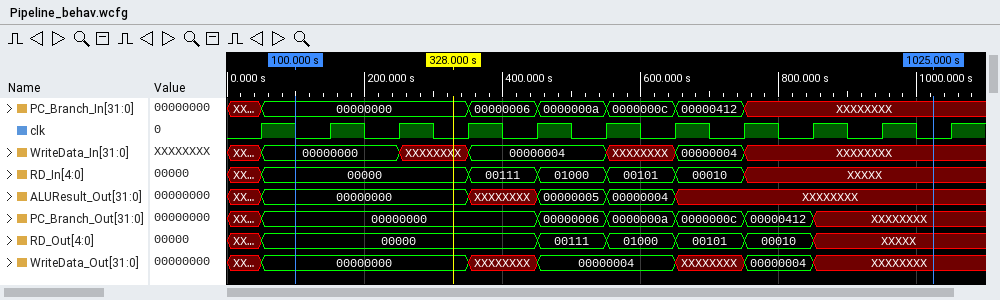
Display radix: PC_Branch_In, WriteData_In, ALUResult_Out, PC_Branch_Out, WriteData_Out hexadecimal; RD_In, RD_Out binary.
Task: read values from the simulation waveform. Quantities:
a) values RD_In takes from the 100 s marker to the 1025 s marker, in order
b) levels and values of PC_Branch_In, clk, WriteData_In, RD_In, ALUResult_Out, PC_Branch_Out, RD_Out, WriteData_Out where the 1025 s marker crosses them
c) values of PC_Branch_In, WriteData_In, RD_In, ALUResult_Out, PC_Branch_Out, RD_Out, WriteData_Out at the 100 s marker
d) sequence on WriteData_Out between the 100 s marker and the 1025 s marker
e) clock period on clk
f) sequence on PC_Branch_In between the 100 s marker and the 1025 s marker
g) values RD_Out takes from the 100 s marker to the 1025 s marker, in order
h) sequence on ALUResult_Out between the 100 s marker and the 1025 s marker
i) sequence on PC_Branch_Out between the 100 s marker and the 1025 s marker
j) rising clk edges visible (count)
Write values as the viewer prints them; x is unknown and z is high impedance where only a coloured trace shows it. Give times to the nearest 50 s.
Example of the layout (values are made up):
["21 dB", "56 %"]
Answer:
["00000, 00111, 01000, 00101, 00010, XXXXX", "PC_Branch_In=XXXXXXXX, clk=0, WriteData_In=XXXXXXXX, RD_In=XXXXX, ALUResult_Out=XXXXXXXX, PC_Branch_Out=XXXXXXXX, RD_Out=XXXXX, WriteData_Out=XXXXXXXX", "PC_Branch_In=00000000, WriteData_In=00000000, RD_In=00000, ALUResult_Out=00000000, PC_Branch_Out=00000000, RD_Out=00000, WriteData_Out=00000000", "00000000, XXXXXXXX, 00000004, XXXXXXXX, 00000004, XXXXXXXX", "100 s", "00000000, 00000006, 0000000a, 0000000c, 00000412, XXXXXXXX", "00000, 00111, 01000, 00101, 00010, XXXXX", "00000000, XXXXXXXX, 00000005, 00000004, XXXXXXXX", "00000000, 00000006, 0000000a, 0000000c, 00000412, XXXXXXXX", "11"]
